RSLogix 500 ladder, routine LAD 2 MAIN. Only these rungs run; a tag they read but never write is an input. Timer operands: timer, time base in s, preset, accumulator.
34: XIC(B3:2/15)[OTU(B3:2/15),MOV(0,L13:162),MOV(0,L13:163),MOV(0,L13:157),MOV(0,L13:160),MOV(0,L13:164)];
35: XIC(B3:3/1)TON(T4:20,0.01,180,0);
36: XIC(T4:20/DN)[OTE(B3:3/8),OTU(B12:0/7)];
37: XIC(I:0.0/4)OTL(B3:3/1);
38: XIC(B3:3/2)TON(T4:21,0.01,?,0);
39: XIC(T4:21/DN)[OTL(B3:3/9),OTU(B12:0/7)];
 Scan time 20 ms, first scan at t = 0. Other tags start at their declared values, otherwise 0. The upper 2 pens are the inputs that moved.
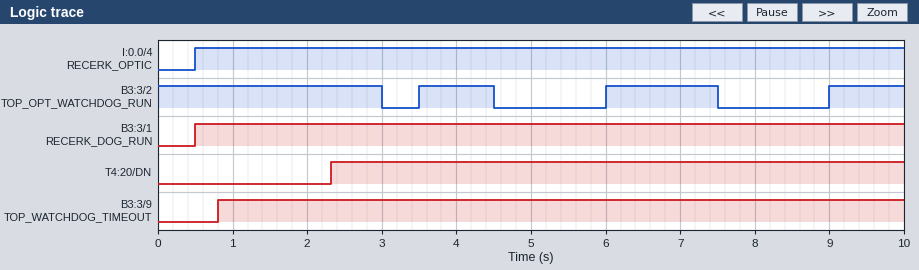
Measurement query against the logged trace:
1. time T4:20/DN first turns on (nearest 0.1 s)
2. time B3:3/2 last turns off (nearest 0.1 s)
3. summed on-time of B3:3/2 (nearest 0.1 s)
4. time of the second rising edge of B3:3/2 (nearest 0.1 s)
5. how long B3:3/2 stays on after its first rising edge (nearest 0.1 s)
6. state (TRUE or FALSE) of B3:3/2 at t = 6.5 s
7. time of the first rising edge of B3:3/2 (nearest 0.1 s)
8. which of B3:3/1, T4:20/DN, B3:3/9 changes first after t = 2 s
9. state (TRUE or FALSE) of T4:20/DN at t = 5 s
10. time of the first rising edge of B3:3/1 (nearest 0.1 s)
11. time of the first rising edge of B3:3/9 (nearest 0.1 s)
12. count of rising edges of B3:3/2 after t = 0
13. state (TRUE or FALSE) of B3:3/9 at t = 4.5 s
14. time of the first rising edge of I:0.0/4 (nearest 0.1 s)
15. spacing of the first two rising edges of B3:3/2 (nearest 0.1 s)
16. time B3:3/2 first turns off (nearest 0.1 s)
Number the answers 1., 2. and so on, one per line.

1. 2.3 s
2. 7.5 s
3. 6.5 s
4. 6.0 s
5. 1.0 s
6. TRUE
7. 3.5 s
8. T4:20/DN
9. TRUE
10. 0.5 s
11. 0.8 s
12. 3
13. TRUE
14. 0.5 s
15. 2.5 s
16. 3.0 s
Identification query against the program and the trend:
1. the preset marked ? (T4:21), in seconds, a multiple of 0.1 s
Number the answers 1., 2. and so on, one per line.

1. 0.8 s
